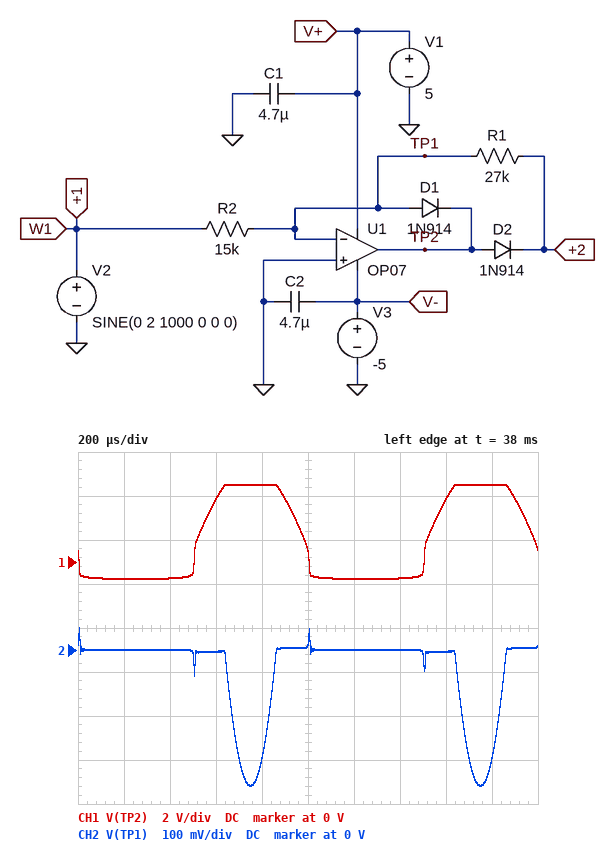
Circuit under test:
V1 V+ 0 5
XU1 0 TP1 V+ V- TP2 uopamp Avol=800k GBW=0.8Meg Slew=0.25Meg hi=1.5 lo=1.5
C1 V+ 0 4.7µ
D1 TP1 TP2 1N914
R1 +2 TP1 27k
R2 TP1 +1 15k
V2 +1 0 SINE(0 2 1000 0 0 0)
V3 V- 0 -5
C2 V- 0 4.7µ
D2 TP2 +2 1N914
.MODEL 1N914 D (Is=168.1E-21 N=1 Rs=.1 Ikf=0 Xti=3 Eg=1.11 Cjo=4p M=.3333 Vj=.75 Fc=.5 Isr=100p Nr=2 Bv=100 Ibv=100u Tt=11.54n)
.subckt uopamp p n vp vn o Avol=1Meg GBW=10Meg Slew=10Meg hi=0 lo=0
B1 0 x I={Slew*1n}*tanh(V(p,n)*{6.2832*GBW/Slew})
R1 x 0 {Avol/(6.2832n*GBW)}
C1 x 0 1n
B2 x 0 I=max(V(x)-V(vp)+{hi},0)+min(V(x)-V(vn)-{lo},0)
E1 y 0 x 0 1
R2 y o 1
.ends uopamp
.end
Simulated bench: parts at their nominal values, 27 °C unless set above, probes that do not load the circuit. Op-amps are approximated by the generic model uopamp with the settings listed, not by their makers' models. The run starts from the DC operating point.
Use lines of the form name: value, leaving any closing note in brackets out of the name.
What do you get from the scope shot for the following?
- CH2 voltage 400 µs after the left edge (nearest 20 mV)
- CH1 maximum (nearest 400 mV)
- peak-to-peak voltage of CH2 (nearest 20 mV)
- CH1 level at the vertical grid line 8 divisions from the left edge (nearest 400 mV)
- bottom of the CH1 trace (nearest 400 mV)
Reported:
CH2 voltage 400 µs after the left edge: 0 V
CH1 maximum: 3.6 V
peak-to-peak voltage of CH2: 360 mV
CH1 level at the vertical grid line 8 divisions from the left edge: 2.8 V
bottom of the CH1 trace: -800 mV
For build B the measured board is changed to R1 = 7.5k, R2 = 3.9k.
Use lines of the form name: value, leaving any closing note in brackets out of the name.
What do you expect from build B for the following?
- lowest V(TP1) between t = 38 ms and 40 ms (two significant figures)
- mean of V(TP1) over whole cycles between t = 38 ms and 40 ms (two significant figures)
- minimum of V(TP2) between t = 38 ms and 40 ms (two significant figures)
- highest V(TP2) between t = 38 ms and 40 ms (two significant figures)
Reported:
lowest V(TP1) between t = 38 ms and 40 ms: -400 mV
mean of V(TP1) over whole cycles between t = 38 ms and 40 ms: -67 mV
minimum of V(TP2) between t = 38 ms and 40 ms: -830 mV
highest V(TP2) between t = 38 ms and 40 ms: 3.5 V
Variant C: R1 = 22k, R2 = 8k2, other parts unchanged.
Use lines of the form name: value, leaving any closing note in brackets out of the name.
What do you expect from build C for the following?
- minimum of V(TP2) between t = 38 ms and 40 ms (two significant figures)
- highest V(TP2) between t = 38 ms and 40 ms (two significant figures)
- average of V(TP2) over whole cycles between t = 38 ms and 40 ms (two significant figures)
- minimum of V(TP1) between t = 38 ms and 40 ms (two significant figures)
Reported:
minimum of V(TP2) between t = 38 ms and 40 ms: -800 mV
highest V(TP2) between t = 38 ms and 40 ms: 3.5 V
average of V(TP2) over whole cycles between t = 38 ms and 40 ms: 1.1 V
minimum of V(TP1) between t = 38 ms and 40 ms: -720 mV
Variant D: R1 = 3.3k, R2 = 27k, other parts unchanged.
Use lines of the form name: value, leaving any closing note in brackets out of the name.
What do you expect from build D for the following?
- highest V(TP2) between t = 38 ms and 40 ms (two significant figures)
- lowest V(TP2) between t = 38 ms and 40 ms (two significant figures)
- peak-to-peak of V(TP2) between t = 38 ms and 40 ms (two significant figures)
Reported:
highest V(TP2) between t = 38 ms and 40 ms: 990 mV
lowest V(TP2) between t = 38 ms and 40 ms: -740 mV
peak-to-peak of V(TP2) between t = 38 ms and 40 ms: 1.7 V
